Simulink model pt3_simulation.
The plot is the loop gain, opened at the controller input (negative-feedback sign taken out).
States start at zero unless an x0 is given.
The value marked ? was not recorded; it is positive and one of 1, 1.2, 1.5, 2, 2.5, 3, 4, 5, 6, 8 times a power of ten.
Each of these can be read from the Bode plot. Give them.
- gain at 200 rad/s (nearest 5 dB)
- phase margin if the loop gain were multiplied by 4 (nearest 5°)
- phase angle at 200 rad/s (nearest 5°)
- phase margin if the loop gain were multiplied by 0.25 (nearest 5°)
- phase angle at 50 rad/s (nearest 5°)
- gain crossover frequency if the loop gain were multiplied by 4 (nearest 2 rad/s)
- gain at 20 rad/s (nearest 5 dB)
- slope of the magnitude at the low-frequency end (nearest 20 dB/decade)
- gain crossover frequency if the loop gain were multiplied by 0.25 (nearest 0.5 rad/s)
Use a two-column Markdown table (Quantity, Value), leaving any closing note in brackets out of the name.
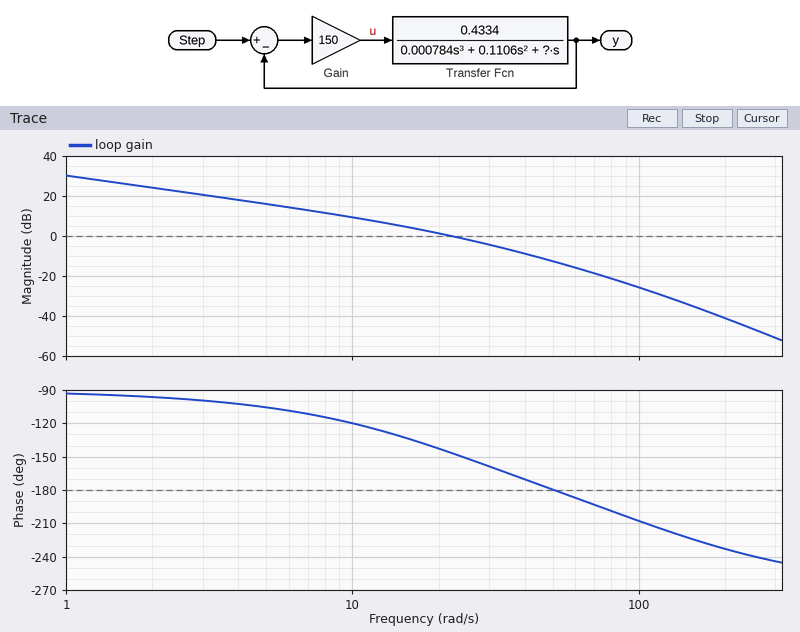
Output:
| Quantity | Value |
|---|---|
| gain at 200 rad/s | -40 dB |
| phase margin if the loop gain were multiplied by 4 | 0° |
| phase angle at 200 rad/s | -235° |
| phase margin if the loop gain were multiplied by 0.25 | 65° |
| phase angle at 50 rad/s | -180° |
| gain crossover frequency if the loop gain were multiplied by 4 | 48 rad/s |
| gain at 20 rad/s | 0 dB |
| slope of the magnitude at the low-frequency end | -20 dB/decade |
| gain crossover frequency if the loop gain were multiplied by 0.25 | 7.5 rad/s |
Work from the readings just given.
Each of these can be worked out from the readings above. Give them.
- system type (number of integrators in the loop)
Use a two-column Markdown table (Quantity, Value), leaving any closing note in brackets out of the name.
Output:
| Quantity | Value |
|---|---|
| system type | 1 |
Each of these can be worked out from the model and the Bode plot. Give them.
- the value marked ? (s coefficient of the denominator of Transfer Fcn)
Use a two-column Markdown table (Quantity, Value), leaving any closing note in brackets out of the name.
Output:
| Quantity | Value |
|---|---|
| the value marked ? | 2 |
